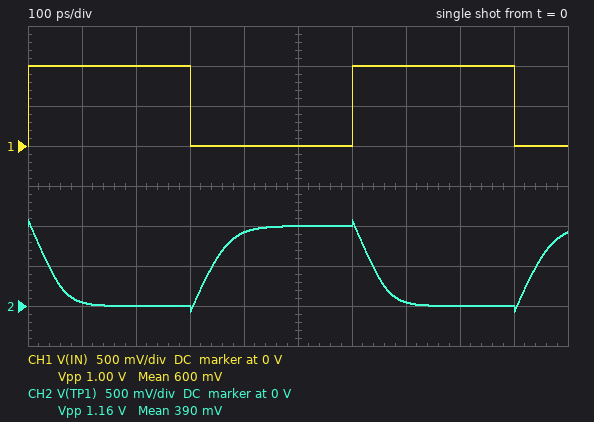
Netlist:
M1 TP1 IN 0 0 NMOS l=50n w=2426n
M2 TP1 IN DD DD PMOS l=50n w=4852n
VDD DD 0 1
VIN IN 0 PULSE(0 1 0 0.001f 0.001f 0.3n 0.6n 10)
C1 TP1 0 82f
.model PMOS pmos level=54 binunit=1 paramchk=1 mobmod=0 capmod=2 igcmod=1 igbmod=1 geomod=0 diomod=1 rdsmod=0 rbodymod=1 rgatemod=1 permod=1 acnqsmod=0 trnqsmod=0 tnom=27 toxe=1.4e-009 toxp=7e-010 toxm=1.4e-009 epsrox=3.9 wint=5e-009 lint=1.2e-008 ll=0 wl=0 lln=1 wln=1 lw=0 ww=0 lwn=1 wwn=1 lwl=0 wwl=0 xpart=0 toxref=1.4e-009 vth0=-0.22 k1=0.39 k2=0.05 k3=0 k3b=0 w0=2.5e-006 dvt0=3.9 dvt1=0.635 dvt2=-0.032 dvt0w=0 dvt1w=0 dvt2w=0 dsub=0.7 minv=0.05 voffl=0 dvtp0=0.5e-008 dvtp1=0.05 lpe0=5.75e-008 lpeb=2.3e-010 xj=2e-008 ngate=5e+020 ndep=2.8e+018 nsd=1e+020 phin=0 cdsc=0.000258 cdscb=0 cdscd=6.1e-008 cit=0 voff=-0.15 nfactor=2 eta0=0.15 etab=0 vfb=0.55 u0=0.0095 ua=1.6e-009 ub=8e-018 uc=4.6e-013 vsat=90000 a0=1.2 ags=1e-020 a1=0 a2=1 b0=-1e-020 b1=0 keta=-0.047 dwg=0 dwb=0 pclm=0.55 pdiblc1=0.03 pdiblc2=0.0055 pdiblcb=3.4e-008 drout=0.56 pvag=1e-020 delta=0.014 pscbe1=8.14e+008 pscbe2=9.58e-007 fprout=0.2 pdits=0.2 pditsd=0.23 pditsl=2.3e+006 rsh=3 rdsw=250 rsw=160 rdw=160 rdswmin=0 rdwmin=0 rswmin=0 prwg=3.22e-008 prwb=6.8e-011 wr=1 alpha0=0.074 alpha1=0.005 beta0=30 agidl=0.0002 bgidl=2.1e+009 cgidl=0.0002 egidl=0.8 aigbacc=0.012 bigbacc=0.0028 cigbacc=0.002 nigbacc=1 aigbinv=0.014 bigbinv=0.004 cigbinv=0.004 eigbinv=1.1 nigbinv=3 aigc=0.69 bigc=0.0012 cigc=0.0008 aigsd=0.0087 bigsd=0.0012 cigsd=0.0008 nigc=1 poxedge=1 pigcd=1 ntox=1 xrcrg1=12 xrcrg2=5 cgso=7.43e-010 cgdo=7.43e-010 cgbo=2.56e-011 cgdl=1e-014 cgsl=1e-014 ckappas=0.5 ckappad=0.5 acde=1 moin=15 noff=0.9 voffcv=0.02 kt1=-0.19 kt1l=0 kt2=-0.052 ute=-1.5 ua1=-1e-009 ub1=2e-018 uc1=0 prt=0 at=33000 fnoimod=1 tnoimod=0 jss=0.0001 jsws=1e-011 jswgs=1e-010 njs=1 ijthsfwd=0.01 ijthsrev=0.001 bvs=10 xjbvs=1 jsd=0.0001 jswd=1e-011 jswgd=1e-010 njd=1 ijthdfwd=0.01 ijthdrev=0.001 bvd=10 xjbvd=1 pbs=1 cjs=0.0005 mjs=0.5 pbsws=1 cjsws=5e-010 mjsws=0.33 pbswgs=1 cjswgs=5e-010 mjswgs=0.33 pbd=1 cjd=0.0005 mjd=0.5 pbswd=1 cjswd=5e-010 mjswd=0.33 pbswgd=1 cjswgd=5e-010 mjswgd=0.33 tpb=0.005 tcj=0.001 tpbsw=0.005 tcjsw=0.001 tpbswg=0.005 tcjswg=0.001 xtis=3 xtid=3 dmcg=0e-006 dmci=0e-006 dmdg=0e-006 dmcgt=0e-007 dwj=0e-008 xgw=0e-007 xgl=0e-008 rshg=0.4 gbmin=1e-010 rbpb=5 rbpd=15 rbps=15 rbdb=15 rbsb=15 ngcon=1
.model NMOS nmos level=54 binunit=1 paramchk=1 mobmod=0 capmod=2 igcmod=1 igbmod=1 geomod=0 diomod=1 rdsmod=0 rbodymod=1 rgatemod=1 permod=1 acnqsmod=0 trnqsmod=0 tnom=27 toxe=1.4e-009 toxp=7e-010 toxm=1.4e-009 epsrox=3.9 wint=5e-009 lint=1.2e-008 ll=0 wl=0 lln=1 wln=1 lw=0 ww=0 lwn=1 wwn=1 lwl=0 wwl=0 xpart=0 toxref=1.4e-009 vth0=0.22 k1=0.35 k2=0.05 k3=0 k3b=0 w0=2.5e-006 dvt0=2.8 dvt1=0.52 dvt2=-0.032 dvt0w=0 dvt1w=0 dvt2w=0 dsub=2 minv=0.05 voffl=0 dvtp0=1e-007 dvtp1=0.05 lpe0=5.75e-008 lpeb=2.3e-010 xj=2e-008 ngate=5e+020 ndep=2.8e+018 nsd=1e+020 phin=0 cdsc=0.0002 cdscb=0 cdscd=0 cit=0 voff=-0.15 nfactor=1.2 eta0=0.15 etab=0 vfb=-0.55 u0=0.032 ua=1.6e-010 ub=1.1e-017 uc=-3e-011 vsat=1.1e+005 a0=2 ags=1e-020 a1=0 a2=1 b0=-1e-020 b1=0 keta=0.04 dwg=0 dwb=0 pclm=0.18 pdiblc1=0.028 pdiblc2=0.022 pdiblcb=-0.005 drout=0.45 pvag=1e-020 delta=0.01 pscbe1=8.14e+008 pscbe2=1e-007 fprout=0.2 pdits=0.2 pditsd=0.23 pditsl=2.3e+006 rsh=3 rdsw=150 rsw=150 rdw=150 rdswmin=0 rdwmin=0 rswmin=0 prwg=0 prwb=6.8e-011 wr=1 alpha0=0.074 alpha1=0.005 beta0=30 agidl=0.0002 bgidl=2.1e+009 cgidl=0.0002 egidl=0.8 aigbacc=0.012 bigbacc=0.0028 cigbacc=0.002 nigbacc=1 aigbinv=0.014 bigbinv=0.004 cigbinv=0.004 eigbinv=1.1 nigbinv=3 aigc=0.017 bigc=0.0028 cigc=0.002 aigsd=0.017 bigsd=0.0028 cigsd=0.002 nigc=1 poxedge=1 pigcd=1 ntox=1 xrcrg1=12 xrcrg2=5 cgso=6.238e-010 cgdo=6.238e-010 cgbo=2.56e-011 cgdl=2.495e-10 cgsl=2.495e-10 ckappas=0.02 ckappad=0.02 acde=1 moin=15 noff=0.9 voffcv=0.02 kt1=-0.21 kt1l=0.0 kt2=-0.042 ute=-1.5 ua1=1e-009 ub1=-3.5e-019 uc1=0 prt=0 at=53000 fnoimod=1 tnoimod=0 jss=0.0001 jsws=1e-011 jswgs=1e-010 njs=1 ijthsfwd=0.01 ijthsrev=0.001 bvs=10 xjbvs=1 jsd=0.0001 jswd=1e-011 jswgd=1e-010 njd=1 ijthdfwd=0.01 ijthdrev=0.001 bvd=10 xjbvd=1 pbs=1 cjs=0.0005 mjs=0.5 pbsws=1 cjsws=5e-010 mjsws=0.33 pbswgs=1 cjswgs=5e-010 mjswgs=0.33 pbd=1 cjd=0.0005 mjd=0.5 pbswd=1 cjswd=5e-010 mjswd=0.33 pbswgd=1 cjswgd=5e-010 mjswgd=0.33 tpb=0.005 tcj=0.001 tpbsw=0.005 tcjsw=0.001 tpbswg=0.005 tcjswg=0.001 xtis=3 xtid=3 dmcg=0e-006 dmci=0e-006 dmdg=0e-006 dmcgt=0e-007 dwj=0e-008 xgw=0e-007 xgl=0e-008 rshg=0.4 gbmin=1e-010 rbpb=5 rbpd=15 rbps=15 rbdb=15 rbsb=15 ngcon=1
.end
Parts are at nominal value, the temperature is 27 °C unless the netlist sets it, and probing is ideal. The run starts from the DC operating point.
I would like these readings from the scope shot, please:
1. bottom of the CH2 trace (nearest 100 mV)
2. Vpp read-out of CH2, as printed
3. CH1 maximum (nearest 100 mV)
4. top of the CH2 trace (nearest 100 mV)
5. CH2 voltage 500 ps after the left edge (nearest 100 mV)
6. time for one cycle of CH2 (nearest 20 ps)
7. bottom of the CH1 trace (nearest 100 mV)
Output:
-100 mV
1.16 V
1.0 V
1.1 V
1.0 V
600 ps
0 V
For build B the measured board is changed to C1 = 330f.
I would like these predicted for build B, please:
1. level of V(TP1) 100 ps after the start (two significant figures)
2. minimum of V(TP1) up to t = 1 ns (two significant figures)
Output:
600 mV
38 mV
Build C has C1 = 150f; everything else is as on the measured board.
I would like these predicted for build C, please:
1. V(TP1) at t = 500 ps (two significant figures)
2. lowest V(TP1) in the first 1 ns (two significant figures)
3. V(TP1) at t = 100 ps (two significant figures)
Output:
960 mV
-44 mV
240 mV
